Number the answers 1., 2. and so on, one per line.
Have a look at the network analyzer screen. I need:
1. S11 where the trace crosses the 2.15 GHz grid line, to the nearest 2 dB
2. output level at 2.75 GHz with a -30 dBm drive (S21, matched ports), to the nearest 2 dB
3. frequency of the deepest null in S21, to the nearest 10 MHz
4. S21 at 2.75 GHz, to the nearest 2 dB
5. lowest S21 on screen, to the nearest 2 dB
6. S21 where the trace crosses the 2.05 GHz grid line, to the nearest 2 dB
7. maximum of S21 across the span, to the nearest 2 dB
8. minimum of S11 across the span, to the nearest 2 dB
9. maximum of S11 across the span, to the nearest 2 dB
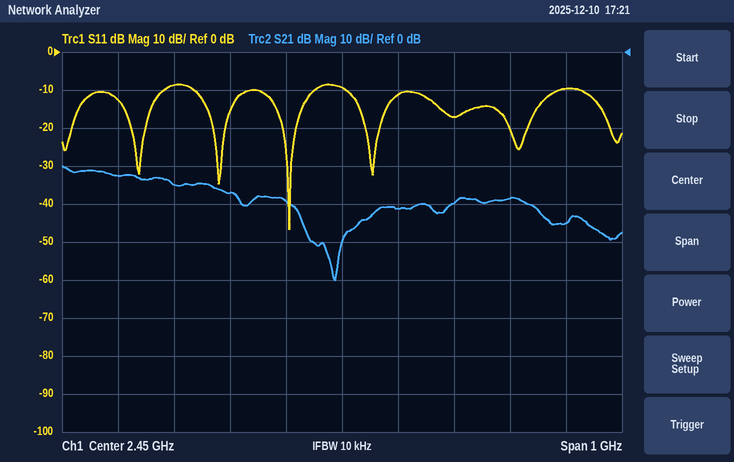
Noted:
1. -8 dB
2. -68 dBm
3. 2.44 GHz
4. -38 dB
5. -60 dB
6. -32 dB
7. -30 dB
8. -46 dB
9. -8 dB
